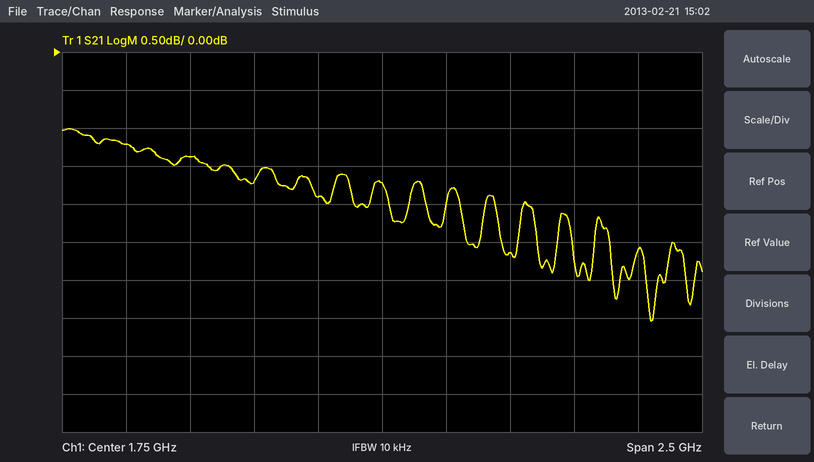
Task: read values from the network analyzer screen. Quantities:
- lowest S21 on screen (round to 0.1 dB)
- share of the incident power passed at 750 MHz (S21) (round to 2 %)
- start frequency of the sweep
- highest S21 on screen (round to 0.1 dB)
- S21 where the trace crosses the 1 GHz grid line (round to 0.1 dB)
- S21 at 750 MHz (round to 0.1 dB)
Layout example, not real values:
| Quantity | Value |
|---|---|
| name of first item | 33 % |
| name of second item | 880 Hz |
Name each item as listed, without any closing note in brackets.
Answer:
| Quantity | Value |
|---|---|
| lowest S21 on screen | -3.5 dB |
| share of the incident power passed at 750 MHz (S21) | 76 % |
| start frequency of the sweep | 500 MHz |
| highest S21 on screen | -1.0 dB |
| S21 where the trace crosses the 1 GHz grid line | -1.4 dB |
| S21 at 750 MHz | -1.2 dB |
